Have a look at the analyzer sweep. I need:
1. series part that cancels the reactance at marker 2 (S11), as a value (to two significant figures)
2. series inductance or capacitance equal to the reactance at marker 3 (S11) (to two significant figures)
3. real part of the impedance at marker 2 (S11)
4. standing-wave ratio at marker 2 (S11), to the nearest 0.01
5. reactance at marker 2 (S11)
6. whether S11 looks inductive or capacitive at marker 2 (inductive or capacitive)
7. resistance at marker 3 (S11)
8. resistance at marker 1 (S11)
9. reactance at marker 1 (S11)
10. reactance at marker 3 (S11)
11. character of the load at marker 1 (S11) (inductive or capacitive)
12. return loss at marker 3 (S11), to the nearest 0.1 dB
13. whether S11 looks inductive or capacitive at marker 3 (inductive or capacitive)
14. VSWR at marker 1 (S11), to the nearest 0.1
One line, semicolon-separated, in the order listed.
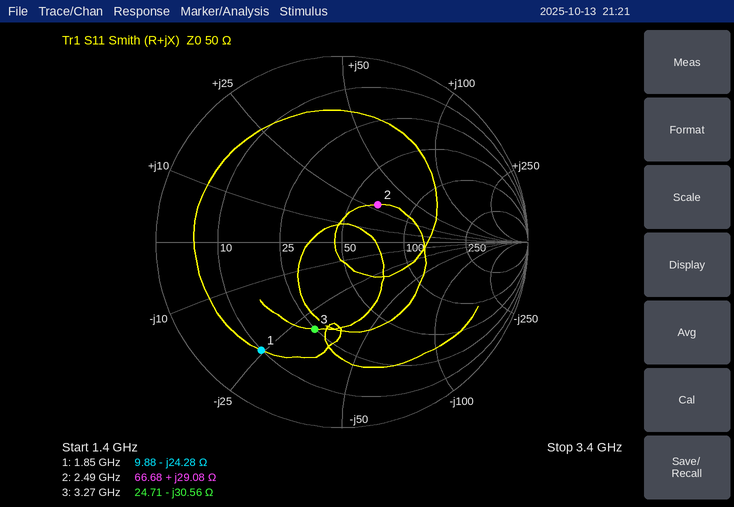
2.2 pF; 1.6 pF; 66.68 Ω; 1.77; +29.08 Ω; inductive; 24.71 Ω; 9.88 Ω; -24.28 Ω; -30.56 Ω; capacitive; 6.2 dB; capacitive; 6.3
